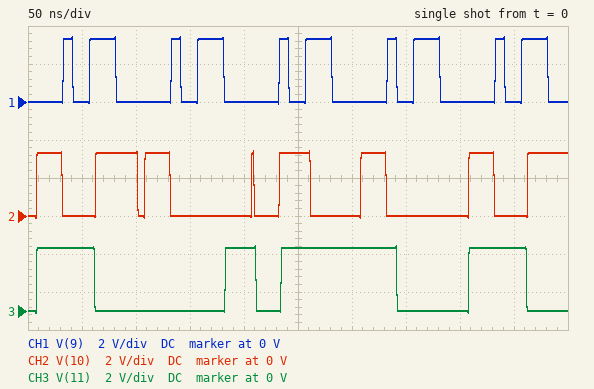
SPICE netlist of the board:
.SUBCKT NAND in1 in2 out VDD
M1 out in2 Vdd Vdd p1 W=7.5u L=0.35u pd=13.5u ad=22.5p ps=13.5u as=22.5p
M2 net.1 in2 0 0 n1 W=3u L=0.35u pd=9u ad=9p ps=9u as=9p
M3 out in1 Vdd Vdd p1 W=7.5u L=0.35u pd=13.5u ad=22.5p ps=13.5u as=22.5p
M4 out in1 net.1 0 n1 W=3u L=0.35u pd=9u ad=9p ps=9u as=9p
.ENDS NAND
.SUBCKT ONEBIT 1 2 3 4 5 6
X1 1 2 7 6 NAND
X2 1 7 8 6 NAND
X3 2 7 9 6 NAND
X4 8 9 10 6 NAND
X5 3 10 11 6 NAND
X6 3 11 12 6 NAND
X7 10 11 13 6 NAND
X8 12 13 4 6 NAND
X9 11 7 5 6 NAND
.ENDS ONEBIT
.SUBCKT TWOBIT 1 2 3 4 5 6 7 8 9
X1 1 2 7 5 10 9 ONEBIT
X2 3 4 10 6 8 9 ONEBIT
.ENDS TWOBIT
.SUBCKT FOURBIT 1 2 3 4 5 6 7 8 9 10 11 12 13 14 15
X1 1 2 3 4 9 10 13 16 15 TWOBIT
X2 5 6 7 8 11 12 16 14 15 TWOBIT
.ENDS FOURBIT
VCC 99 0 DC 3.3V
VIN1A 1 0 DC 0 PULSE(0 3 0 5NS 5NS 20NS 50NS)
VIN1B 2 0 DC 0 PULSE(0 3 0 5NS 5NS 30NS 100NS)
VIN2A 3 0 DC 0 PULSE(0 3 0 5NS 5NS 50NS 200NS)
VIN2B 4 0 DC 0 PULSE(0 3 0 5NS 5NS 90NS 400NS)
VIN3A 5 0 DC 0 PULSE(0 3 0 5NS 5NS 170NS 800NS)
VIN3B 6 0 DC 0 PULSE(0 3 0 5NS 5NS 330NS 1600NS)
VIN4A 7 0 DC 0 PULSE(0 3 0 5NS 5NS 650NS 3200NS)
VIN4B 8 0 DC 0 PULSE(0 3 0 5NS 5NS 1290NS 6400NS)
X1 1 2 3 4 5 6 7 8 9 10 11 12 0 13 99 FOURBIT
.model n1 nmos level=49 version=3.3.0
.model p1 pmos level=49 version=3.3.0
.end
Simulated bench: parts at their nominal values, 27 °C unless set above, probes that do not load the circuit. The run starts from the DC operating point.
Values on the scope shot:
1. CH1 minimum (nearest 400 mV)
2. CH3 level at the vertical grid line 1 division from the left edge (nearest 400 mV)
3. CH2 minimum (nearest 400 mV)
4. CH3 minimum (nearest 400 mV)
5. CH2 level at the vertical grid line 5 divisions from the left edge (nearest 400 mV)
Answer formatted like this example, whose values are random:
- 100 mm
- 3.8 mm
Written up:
- 0 V
- 3.2 V
- 0 V
- 0 V
- 3.2 V
